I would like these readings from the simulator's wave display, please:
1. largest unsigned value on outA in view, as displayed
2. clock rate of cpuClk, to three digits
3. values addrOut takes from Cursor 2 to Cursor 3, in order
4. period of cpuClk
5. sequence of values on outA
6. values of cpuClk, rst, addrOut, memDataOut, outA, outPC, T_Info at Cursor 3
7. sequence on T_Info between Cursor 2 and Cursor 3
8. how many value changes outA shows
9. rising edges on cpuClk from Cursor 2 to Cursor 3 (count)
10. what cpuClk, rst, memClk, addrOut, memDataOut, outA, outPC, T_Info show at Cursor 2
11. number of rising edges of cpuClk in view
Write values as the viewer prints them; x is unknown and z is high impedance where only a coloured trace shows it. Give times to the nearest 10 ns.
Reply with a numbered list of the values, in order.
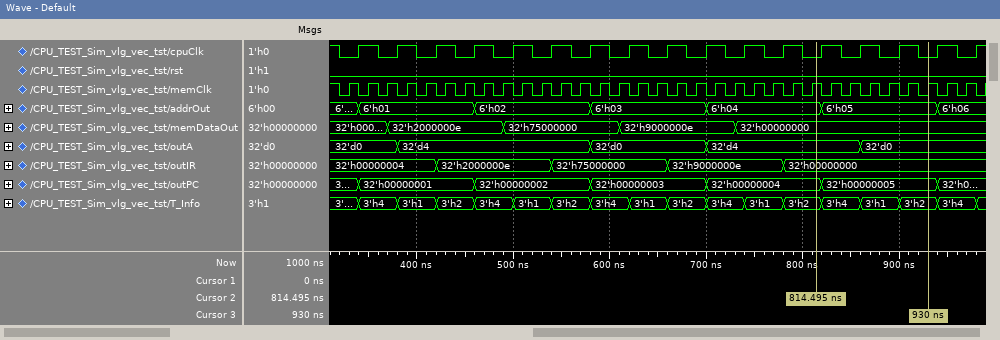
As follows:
1. 32'd4
2. 25.0 MHz
3. 6'h04, 6'h05
4. 40 ns
5. 32'd0, 32'd4, 32'd0, 32'd4, 32'd0
6. cpuClk=0, rst=0, addrOut=6'h05, memDataOut=32'h00000000, outA=32'd0, outPC=32'h00000005, T_Info=3'h2
7. 3'h2, 3'h4, 3'h1, 3'h2
8. 4
9. 3
10. cpuClk=0, rst=0, memClk=1, addrOut=6'h04, memDataOut=32'h00000000, outA=32'd4, outPC=32'h00000004, T_Info=3'h2
11. 17
